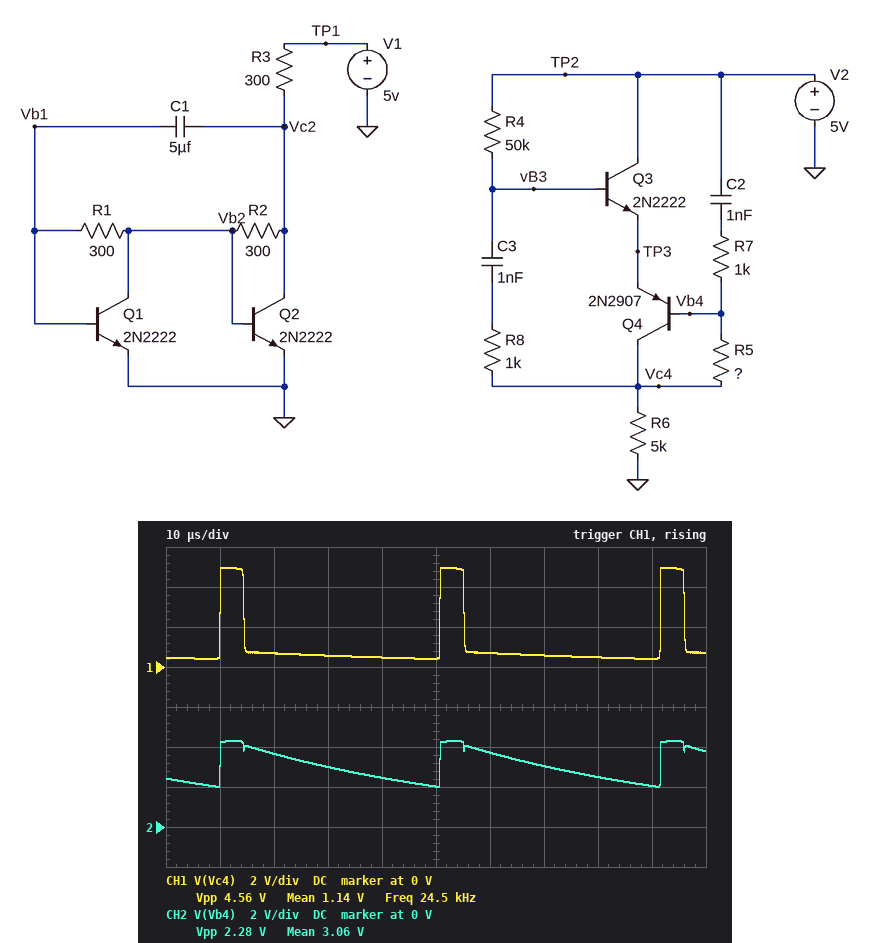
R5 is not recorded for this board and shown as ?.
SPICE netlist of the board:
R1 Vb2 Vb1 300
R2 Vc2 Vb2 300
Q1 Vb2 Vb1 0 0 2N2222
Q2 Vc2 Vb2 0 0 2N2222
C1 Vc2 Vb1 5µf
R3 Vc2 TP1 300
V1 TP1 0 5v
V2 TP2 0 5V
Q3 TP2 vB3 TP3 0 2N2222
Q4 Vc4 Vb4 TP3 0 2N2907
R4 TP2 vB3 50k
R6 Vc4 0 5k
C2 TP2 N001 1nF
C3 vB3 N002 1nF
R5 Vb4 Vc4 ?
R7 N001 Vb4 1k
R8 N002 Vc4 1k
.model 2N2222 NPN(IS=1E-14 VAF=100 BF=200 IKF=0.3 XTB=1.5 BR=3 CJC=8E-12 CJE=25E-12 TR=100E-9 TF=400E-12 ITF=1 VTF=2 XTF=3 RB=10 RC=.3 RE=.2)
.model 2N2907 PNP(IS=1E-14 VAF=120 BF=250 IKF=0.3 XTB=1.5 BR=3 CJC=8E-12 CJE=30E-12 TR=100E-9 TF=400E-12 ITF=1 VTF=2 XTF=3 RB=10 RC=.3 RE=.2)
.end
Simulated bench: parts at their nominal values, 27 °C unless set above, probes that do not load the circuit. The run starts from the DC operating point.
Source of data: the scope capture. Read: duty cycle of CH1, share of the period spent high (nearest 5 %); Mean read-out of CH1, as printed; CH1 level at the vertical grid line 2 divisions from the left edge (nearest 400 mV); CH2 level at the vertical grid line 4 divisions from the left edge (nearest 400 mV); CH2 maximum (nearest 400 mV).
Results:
10 %
1.14 V
800 mV
2.4 V
4.4 V
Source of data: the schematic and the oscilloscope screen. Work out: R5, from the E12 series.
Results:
39 kΩ
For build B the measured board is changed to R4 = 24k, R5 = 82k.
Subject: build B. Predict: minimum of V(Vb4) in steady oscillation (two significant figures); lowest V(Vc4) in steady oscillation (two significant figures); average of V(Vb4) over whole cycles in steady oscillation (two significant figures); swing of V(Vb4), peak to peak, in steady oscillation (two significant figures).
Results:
2.9 V
380 mV
3.6 V
1.4 V
